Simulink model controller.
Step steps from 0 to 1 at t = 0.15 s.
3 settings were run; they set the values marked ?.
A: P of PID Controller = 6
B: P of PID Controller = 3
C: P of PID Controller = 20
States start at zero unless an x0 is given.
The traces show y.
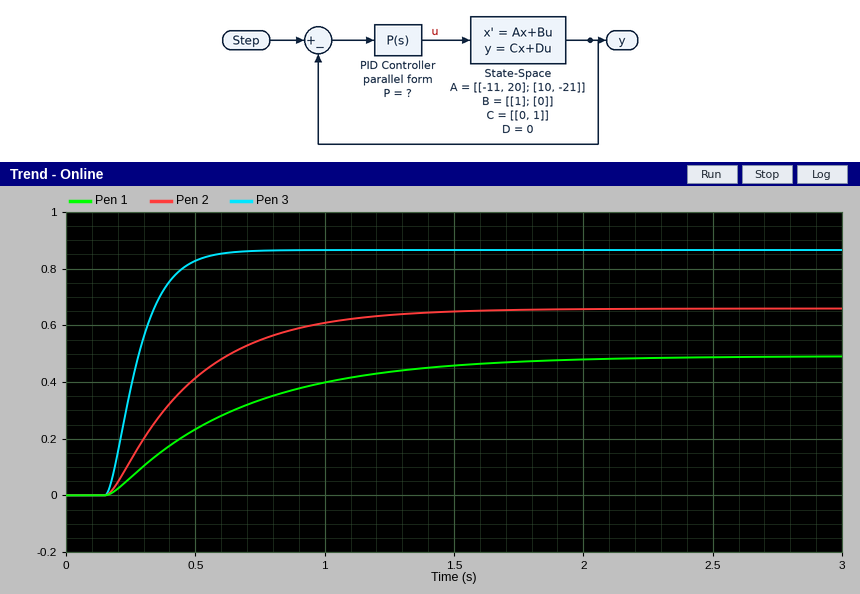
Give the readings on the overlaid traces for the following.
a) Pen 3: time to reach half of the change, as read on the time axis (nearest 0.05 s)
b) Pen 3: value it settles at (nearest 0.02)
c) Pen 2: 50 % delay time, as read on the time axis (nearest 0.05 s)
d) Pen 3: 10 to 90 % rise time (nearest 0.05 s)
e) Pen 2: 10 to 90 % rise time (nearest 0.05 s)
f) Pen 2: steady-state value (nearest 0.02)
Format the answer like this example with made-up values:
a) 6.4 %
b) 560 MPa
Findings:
a) 0.25 s
b) 0.86
c) 0.40 s
d) 0.25 s
e) 0.70 s
f) 0.66
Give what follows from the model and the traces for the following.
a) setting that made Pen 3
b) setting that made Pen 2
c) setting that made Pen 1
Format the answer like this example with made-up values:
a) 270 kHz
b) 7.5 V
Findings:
a) C
b) A
c) B
